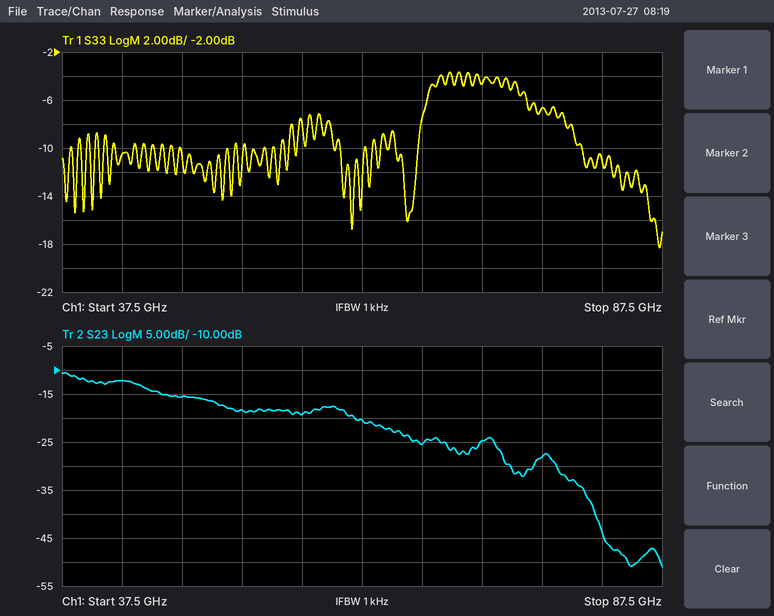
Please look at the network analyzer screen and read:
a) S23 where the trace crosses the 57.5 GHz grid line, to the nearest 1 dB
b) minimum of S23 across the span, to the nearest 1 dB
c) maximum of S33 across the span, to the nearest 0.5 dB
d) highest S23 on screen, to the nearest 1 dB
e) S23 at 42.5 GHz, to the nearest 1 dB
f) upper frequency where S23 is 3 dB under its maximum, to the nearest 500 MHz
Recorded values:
-19 dB
-51 dB
-3.5 dB
-11 dB
-12 dB
44.5 GHz
